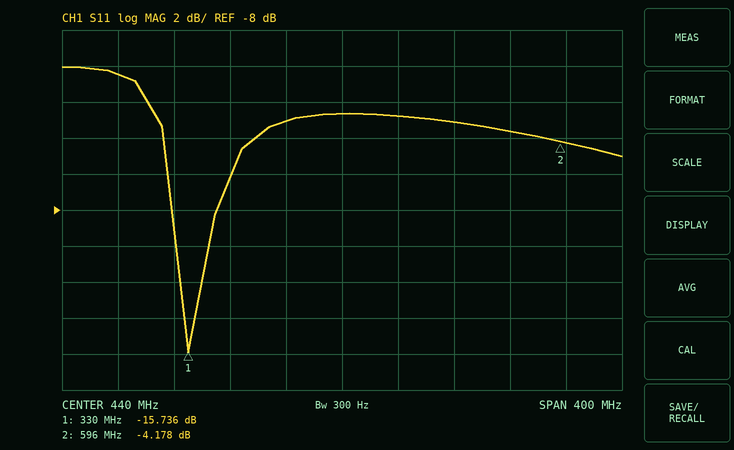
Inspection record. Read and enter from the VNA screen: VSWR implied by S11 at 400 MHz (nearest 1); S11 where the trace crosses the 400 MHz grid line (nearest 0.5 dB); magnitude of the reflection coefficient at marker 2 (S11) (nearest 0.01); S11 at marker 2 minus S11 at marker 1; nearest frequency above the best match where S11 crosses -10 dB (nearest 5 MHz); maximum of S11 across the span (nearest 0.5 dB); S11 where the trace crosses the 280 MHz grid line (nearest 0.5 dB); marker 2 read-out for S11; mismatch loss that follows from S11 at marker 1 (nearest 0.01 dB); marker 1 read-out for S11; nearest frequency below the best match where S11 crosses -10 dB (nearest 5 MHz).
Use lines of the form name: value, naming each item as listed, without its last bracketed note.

VSWR implied by S11 at 400 MHz: 6
S11 where the trace crosses the 400 MHz grid line: -3.0 dB
magnitude of the reflection coefficient at marker 2 (S11): 0.62
S11 at marker 2 minus S11 at marker 1: 11.558 dB
nearest frequency above the best match where S11 crosses -10 dB: 345 MHz
maximum of S11 across the span: 0.0 dB
S11 where the trace crosses the 280 MHz grid line: -0.5 dB
marker 2 read-out for S11: -4.178 dB
mismatch loss that follows from S11 at marker 1: 0.12 dB
marker 1 read-out for S11: -15.736 dB
nearest frequency below the best match where S11 crosses -10 dB: 320 MHz
